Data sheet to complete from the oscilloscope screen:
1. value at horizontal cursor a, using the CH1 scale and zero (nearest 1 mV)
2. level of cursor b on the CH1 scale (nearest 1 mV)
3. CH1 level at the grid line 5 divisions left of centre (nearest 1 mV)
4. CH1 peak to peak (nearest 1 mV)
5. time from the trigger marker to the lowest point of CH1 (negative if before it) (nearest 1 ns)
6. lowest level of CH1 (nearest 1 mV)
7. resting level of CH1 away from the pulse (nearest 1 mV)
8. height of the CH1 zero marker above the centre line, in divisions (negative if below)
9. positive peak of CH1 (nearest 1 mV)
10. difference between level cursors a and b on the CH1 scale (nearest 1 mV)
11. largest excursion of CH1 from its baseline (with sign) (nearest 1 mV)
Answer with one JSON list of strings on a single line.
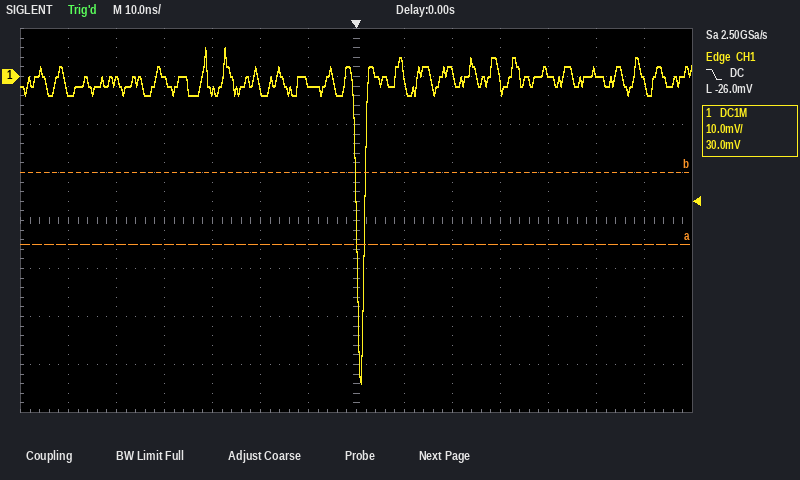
["-35 mV", "-20 mV", "-1 mV", "70 mV", "+1 ns", "-64 mV", "-1 mV", "+3.0 div", "6 mV", "15 mV", "-63 mV"]
